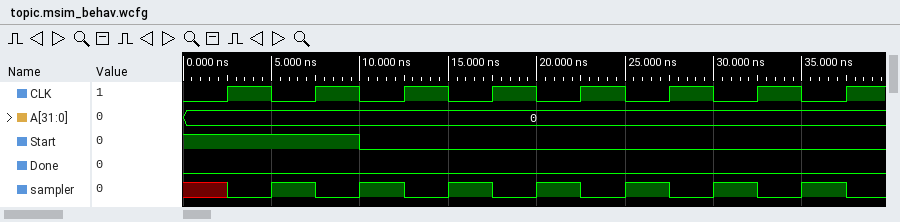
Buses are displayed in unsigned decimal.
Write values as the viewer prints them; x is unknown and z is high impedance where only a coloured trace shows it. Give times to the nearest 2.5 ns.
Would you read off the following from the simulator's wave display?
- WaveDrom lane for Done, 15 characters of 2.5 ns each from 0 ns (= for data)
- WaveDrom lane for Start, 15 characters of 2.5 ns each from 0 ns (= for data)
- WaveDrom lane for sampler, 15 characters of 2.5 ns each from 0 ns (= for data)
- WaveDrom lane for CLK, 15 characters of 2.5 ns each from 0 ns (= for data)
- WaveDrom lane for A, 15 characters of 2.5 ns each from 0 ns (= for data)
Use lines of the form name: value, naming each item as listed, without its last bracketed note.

WaveDrom lane for Done, 15 characters of 2.5 ns each from 0 ns: {name: 'Done', wave: '0..............'}
WaveDrom lane for Start, 15 characters of 2.5 ns each from 0 ns: {name: 'Start', wave: '1...0..........'}
WaveDrom lane for sampler, 15 characters of 2.5 ns each from 0 ns: {name: 'sampler', wave: 'x01010101010101'}
WaveDrom lane for CLK, 15 characters of 2.5 ns each from 0 ns: {name: 'CLK', wave: '010101010101010'}
WaveDrom lane for A, 15 characters of 2.5 ns each from 0 ns: {name: 'A', wave: '=..............', data: '0'}
